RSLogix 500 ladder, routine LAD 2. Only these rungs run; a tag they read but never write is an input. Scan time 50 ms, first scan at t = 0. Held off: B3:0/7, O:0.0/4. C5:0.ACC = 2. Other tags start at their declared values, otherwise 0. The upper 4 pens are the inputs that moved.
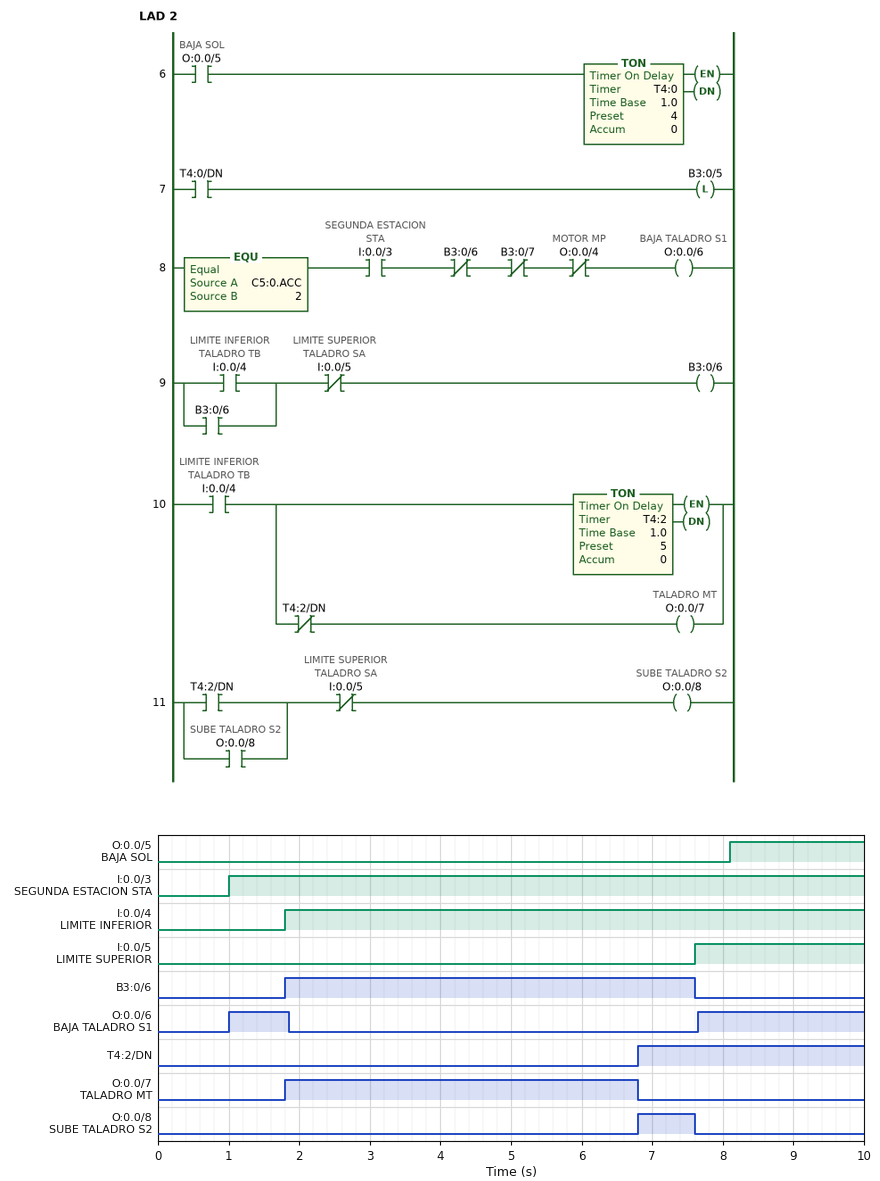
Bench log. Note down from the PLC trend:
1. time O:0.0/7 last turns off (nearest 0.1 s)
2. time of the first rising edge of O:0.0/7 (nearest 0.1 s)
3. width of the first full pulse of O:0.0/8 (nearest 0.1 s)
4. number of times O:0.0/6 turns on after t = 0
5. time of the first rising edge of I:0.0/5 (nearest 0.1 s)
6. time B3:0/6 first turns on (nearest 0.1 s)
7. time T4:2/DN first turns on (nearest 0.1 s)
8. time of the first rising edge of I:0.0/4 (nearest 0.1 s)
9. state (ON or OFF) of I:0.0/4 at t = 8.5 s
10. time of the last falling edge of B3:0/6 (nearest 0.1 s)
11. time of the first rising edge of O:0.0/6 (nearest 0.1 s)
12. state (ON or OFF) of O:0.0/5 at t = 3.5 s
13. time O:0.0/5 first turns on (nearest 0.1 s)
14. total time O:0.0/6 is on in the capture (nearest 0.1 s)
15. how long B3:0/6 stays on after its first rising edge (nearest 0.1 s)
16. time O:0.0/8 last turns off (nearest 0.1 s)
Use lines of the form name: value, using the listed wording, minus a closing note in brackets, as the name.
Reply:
time O:0.0/7 last turns off: 6.8 s
time of the first rising edge of O:0.0/7: 1.8 s
width of the first full pulse of O:0.0/8: 0.8 s
number of times O:0.0/6 turns on after t = 0: 2
time of the first rising edge of I:0.0/5: 7.6 s
time B3:0/6 first turns on: 1.8 s
time T4:2/DN first turns on: 6.8 s
time of the first rising edge of I:0.0/4: 1.8 s
state (ON or OFF) of I:0.0/4 at t = 8.5 s: ON
time of the last falling edge of B3:0/6: 7.6 s
time of the first rising edge of O:0.0/6: 1.0 s
state (ON or OFF) of O:0.0/5 at t = 3.5 s: OFF
time O:0.0/5 first turns on: 8.1 s
total time O:0.0/6 is on in the capture: 3.2 s
how long B3:0/6 stays on after its first rising edge: 5.8 s
time O:0.0/8 last turns off: 7.6 s
